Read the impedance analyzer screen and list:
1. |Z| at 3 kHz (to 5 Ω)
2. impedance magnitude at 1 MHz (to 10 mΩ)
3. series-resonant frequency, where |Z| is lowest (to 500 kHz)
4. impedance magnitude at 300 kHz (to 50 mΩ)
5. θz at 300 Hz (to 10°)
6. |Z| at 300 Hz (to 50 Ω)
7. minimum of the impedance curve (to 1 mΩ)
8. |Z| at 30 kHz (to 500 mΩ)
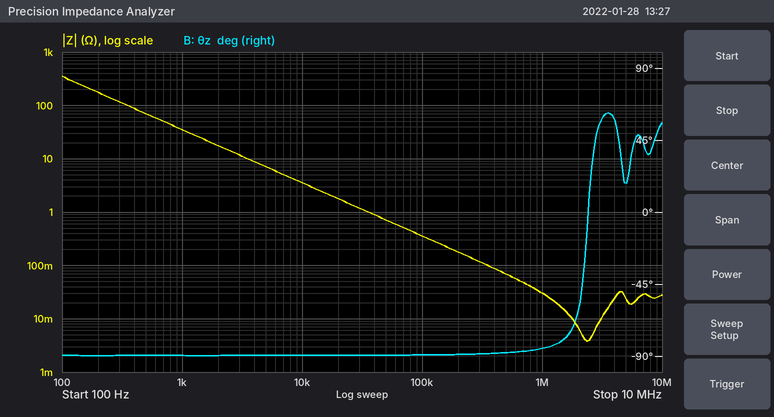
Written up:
10 Ω
30 mΩ
2.5 MHz
100 mΩ
-90°
100 Ω
4 mΩ
1.0 Ω
